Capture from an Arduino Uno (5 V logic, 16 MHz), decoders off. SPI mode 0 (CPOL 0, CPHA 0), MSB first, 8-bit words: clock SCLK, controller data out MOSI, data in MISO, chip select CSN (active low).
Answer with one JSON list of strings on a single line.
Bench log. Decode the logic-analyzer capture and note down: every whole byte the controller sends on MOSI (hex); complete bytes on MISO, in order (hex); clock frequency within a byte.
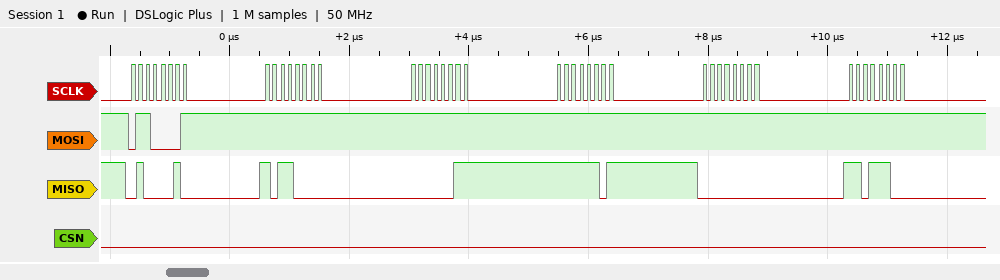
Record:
["0x61 0xFF 0xFF 0xFF 0xFF 0xFF", "0x42 0xB0 0x03 0xFD 0x00 0xDC", "8 MHz"]
